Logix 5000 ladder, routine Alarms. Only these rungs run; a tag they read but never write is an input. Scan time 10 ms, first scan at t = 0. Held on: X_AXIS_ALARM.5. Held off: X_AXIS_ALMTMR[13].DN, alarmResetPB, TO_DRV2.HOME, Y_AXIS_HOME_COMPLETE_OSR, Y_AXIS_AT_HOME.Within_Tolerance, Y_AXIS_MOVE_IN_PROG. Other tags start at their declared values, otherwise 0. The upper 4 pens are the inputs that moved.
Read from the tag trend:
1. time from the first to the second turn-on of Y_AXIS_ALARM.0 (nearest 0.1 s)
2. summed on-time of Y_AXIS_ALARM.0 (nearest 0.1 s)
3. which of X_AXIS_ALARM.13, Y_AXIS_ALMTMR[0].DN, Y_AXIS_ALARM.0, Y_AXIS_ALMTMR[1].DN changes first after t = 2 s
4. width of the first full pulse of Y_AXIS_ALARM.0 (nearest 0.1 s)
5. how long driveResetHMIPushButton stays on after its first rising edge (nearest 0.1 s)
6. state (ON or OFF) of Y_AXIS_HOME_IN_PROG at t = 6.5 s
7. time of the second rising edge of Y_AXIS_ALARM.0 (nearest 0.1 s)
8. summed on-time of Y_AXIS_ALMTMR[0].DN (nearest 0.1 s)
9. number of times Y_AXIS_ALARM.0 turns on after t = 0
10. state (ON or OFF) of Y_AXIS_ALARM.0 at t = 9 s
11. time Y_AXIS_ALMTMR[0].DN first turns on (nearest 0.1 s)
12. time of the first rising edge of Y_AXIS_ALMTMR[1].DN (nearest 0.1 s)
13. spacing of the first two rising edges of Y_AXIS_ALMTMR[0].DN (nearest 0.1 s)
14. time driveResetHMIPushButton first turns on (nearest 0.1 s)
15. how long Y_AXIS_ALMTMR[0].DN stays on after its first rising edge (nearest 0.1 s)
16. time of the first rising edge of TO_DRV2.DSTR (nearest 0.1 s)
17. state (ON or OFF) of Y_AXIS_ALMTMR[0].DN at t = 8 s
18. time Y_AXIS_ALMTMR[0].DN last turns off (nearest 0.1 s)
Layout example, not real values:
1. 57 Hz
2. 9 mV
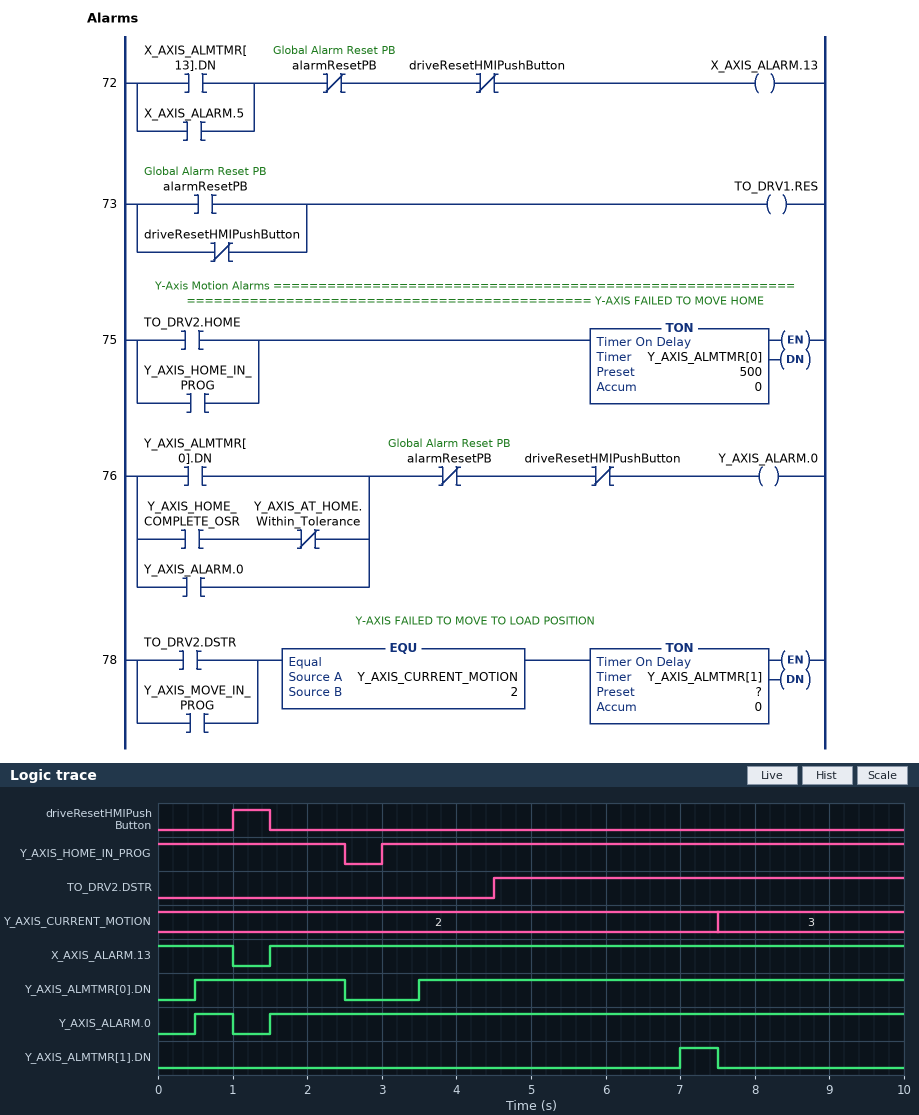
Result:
1. 1.0 s
2. 9.0 s
3. Y_AXIS_ALMTMR[0].DN
4. 0.5 s
5. 0.5 s
6. ON
7. 1.5 s
8. 8.5 s
9. 2
10. ON
11. 0.5 s
12. 7.0 s
13. 3.0 s
14. 1.0 s
15. 2.0 s
16. 4.5 s
17. ON
18. 2.5 s
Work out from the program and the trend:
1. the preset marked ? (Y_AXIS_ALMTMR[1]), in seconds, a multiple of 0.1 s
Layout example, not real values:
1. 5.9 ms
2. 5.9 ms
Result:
1. 2.5 s
